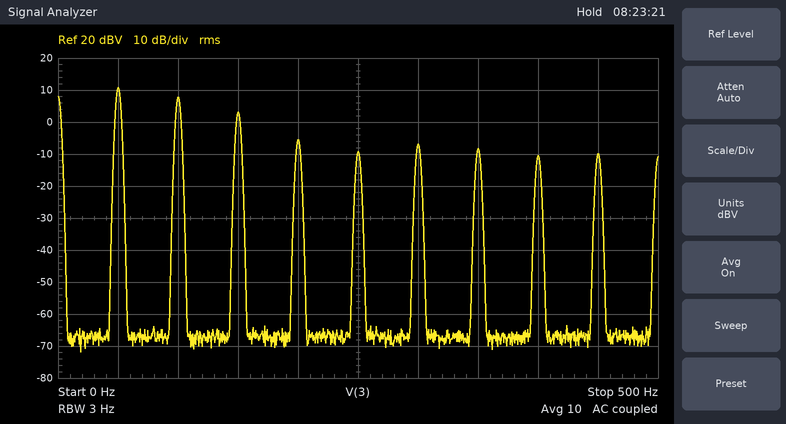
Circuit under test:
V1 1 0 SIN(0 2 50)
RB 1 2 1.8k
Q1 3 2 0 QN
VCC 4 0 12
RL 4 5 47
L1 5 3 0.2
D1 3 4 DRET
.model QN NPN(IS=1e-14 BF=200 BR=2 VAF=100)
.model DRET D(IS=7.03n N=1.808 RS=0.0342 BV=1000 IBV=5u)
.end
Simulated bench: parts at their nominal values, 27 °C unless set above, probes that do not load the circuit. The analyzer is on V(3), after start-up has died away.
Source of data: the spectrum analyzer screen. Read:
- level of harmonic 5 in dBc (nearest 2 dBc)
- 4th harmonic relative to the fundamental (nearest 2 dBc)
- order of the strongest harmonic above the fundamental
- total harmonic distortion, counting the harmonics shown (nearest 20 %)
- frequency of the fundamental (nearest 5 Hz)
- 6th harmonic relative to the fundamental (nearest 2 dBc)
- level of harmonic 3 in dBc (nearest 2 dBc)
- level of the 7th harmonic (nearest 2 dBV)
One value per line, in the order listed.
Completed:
-20 dBc
-16 dBc
2
80 %
50 Hz
-18 dBc
-8 dBc
-8 dBV
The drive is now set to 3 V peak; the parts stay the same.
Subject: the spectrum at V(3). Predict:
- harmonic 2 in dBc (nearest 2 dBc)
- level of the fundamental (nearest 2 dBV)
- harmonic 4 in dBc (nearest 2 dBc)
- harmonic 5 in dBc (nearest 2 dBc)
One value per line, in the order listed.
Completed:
-6 dBc
14 dBV
-14 dBc
-14 dBc
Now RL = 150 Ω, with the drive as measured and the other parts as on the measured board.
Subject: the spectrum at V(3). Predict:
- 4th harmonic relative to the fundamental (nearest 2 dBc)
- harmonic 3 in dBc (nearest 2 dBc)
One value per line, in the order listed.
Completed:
-12 dBc
-26 dBc
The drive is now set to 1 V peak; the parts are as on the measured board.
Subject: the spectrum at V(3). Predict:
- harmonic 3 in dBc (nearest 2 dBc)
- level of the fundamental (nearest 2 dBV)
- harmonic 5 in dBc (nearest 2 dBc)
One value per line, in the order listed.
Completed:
-2 dBc
-4 dBV
-8 dBc
